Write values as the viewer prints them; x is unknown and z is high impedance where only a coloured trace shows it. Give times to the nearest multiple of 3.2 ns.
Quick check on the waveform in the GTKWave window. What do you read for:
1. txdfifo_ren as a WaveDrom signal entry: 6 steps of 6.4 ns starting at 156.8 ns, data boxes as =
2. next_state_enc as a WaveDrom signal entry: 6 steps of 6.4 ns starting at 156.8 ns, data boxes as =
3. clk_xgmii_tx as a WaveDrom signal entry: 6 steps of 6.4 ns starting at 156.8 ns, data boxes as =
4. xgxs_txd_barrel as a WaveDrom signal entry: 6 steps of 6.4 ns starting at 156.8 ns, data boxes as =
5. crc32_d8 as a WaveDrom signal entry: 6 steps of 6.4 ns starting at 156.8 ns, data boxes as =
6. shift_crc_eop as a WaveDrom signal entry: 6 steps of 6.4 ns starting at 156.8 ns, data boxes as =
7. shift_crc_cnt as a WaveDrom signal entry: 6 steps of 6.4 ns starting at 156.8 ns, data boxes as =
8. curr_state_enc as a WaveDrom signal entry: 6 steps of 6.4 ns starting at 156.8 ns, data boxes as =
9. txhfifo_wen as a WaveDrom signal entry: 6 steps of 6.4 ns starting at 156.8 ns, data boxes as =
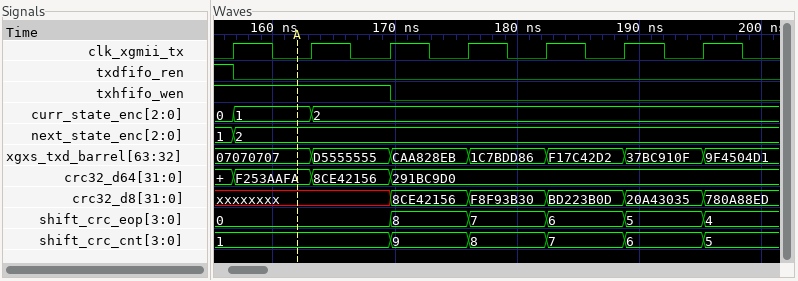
{name: 'txdfifo_ren', wave: '0.....'}
{name: 'next_state_enc', wave: '=.....', data: '2'}
{name: 'clk_xgmii_tx', wave: 'p.....'}
{name: 'xgxs_txd_barrel', wave: '======', data: '07070707 D5555555 CAA828EB 1C7BDD86 F17C42D2 37BC910F'}
{name: 'crc32_d8', wave: 'x.====', data: '8CE42156 F8F93B30 BD223B0D 20A43035'}
{name: 'shift_crc_eop', wave: '=.====', data: '0 8 7 6 5'}
{name: 'shift_crc_cnt', wave: '=.====', data: '1 9 8 7 6'}
{name: 'curr_state_enc', wave: '==....', data: '1 2'}
{name: 'txhfifo_wen', wave: '1.0...'}
